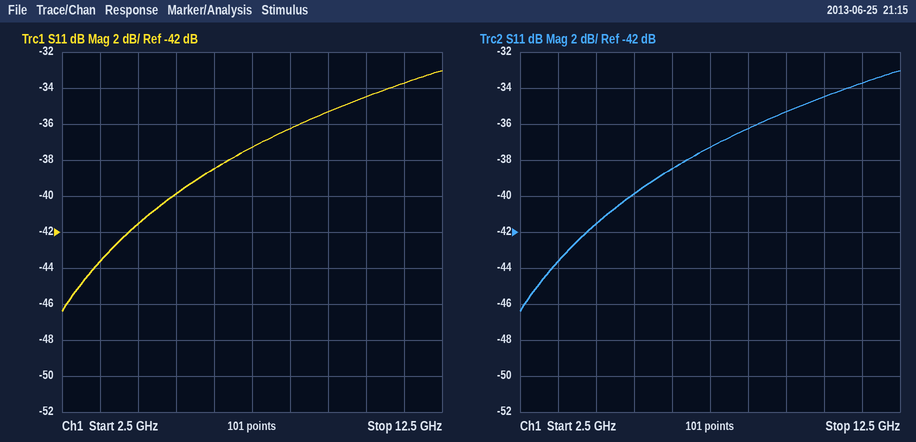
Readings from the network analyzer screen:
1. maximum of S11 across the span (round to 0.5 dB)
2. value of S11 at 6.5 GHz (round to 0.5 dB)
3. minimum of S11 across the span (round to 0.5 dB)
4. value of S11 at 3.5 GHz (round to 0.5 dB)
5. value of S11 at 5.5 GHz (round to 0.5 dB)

-33.0 dB
-38.5 dB
-46.5 dB
-43.5 dB
-40.0 dB
